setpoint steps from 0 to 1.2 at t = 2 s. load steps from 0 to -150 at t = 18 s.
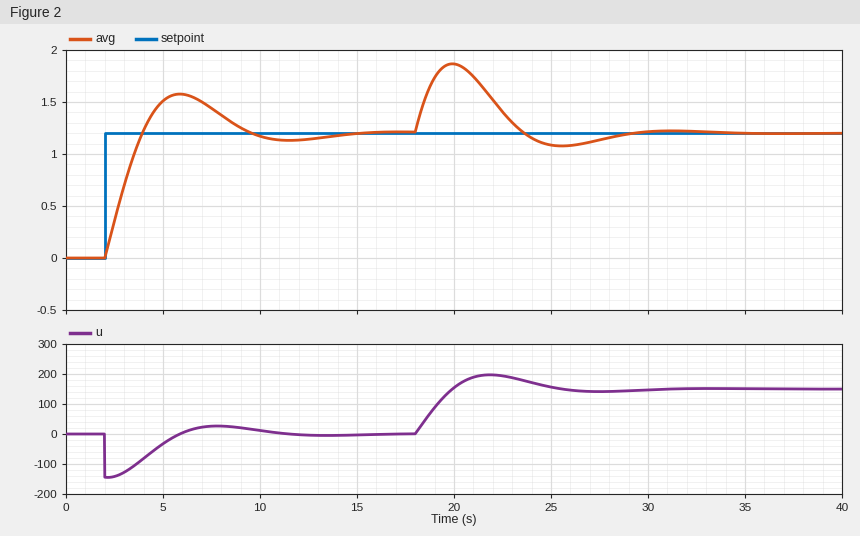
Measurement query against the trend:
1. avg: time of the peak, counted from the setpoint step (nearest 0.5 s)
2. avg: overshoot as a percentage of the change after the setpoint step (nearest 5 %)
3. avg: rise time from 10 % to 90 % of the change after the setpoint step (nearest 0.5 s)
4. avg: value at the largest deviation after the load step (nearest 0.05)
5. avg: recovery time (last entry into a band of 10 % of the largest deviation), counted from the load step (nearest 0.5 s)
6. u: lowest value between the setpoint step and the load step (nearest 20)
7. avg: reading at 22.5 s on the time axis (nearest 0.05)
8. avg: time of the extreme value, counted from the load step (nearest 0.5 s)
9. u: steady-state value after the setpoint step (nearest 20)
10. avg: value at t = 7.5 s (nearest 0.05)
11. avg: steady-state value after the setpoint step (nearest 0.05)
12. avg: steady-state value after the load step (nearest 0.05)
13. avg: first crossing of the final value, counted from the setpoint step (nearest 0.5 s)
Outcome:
4.0 s
30 %
1.5 s
1.85
9.5 s
-140
1.40
2.0 s
0
1.45
1.20
1.20
2.0 s
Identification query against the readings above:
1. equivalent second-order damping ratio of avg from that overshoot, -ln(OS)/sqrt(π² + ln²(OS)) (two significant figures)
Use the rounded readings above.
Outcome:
0.36
